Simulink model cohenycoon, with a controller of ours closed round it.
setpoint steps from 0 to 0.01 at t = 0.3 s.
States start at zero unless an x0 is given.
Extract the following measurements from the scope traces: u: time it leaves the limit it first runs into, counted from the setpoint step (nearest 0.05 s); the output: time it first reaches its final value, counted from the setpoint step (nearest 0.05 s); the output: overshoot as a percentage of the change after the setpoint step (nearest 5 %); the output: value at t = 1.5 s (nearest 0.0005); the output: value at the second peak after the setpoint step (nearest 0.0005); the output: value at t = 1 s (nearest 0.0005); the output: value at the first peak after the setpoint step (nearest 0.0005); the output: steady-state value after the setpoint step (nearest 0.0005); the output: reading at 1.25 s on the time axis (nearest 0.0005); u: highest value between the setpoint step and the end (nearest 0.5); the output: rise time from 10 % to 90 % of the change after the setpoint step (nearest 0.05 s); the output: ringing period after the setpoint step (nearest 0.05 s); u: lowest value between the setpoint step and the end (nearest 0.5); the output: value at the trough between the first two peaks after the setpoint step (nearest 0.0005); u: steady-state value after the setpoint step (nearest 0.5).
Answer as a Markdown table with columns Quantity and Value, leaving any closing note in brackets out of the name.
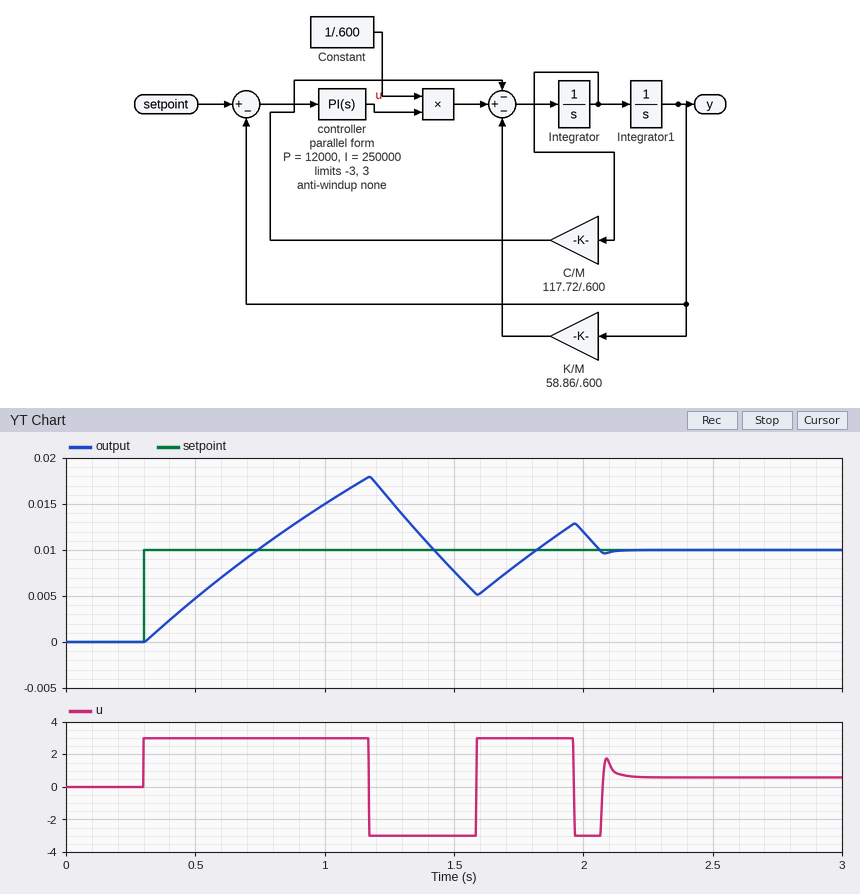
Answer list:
| Quantity | Value |
|---|---|
| u: time it leaves the limit it first runs into, counted from the setpoint step | 0.85 s |
| the output: time it first reaches its final value, counted from the setpoint step | 0.45 s |
| the output: overshoot as a percentage of the change after the setpoint step | 80 % |
| the output: value at t = 1.5 s | 0.0075 |
| the output: value at the second peak after the setpoint step | 0.0130 |
| the output: value at t = 1 s | 0.0150 |
| the output: value at the first peak after the setpoint step | 0.0180 |
| the output: steady-state value after the setpoint step | 0.0100 |
| the output: reading at 1.25 s on the time axis | 0.0155 |
| u: highest value between the setpoint step and the end | 3.0 |
| the output: rise time from 10 % to 90 % of the change after the setpoint step | 0.35 s |
| the output: ringing period after the setpoint step | 0.80 s |
| u: lowest value between the setpoint step and the end | -3.0 |
| the output: value at the trough between the first two peaks after the setpoint step | 0.0050 |
| u: steady-state value after the setpoint step | 0.5 |
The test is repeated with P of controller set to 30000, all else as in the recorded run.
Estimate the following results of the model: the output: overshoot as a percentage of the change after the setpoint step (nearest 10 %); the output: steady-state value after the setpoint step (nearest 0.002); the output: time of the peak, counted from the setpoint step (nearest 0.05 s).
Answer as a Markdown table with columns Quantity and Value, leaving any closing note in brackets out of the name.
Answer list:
| Quantity | Value |
|---|---|
| the output: overshoot as a percentage of the change after the setpoint step | 70 % |
| the output: steady-state value after the setpoint step | 0.010 |
| the output: time of the peak, counted from the setpoint step | 0.80 s |
